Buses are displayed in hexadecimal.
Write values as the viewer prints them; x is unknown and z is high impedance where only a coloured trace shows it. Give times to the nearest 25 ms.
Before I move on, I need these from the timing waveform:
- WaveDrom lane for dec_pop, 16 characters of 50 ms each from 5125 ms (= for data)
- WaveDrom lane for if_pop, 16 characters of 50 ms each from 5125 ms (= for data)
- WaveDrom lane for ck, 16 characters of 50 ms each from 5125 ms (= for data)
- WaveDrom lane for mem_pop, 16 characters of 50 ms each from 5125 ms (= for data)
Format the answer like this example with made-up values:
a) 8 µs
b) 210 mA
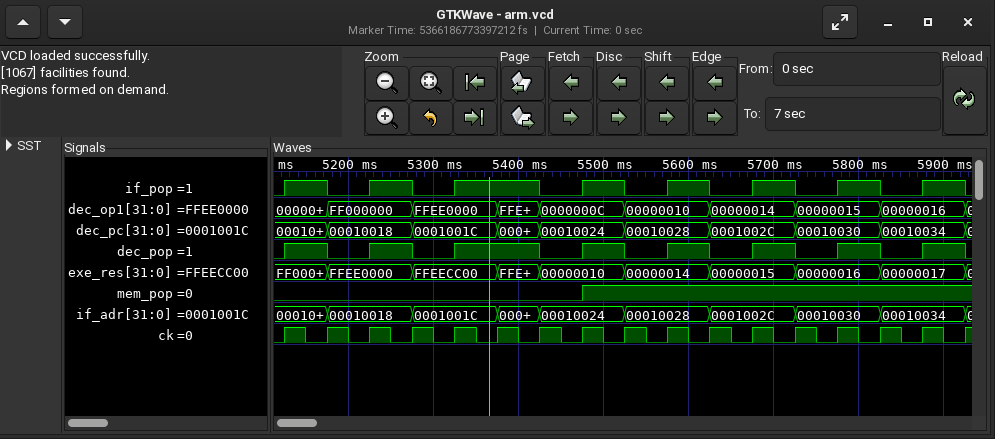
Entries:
a) {name: 'dec_pop', wave: '10101.0101010101'}
b) {name: 'if_pop', wave: '10101.0101010101'}
c) {name: 'ck', wave: 'p...............'}
d) {name: 'mem_pop', wave: '0......1........'}
